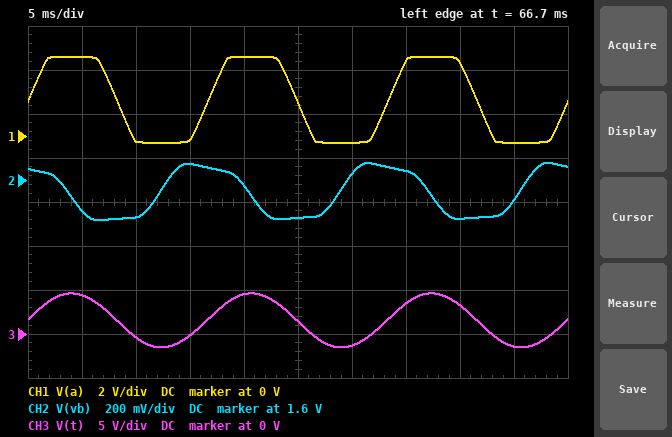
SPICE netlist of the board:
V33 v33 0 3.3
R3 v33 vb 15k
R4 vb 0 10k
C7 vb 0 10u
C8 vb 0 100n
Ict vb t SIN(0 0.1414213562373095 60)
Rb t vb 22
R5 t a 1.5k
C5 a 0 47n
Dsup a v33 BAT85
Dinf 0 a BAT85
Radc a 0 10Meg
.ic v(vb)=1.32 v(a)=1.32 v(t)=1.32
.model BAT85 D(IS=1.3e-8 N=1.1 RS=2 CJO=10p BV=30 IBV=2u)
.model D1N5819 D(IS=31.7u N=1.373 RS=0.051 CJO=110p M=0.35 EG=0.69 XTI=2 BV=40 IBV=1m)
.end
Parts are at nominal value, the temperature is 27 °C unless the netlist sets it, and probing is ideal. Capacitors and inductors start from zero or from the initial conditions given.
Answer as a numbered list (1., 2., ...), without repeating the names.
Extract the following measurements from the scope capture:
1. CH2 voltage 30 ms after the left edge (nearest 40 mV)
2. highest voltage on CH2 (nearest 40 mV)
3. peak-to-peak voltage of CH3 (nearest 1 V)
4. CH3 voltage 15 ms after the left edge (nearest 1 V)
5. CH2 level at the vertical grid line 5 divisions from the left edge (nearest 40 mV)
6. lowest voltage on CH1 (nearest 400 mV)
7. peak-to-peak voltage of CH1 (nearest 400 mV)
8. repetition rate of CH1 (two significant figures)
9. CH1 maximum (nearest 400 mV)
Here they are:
1. 1.64 V
2. 1.68 V
3. 6 V
4. 0 V
5. 1.44 V
6. -400 mV
7. 4.0 V
8. 60 Hz
9. 3.6 V
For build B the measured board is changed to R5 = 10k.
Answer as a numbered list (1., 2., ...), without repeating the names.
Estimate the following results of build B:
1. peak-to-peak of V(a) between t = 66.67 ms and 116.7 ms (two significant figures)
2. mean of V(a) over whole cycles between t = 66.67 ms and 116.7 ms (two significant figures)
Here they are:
1. 3.8 V
2. 1.5 V
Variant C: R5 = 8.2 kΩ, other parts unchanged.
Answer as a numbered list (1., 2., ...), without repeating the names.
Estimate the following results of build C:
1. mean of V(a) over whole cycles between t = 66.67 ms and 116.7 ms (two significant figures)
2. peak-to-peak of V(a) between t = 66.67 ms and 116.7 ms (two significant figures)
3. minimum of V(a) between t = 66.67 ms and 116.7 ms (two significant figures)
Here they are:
1. 1.5 V
2. 3.8 V
3. -270 mV
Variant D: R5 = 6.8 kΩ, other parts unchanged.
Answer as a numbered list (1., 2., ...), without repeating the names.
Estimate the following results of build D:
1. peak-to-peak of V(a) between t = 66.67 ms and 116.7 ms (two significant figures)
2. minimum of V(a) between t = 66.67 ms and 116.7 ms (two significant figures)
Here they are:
1. 3.8 V
2. -280 mV
